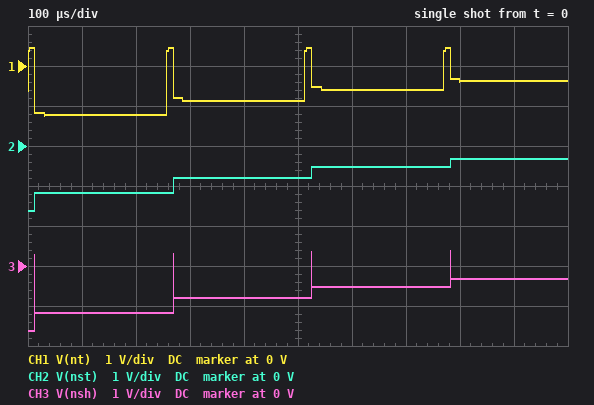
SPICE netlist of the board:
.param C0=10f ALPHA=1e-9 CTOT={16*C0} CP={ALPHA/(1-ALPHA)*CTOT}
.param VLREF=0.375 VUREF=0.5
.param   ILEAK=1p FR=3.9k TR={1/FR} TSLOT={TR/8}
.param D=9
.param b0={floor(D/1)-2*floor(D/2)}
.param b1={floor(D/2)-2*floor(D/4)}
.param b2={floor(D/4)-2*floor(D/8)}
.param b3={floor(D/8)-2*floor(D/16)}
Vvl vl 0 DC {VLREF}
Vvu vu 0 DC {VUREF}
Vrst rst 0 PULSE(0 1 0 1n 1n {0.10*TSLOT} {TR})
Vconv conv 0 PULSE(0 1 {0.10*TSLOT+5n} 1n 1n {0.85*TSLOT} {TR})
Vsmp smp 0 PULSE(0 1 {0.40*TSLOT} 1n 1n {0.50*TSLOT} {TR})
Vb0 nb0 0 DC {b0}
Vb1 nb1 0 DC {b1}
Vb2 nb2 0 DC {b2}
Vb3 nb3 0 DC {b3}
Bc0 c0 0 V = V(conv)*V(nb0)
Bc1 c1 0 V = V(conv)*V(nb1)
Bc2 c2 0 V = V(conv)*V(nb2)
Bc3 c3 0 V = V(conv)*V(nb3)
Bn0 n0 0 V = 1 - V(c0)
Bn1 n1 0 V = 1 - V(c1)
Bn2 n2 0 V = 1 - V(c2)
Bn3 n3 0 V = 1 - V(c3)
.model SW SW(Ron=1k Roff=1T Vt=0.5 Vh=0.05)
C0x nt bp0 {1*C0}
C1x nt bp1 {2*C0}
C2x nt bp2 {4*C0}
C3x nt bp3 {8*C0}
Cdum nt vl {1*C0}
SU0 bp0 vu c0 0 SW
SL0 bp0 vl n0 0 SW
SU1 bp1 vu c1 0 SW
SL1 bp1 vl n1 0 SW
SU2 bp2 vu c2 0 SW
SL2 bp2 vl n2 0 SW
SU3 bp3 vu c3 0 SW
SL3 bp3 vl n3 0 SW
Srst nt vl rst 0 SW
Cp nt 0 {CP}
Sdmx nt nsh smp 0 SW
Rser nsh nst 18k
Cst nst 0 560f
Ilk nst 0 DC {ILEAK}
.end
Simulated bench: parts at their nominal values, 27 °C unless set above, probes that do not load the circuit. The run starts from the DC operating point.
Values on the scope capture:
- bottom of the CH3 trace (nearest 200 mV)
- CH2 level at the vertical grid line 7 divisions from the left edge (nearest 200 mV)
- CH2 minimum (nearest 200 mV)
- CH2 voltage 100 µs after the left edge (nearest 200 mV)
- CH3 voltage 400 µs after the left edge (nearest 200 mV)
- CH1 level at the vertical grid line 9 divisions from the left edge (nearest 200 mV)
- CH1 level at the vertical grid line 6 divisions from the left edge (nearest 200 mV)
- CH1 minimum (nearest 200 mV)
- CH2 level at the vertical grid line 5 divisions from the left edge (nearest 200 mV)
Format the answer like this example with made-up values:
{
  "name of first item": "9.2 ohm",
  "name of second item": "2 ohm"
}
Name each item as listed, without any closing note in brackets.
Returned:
{
  "bottom of the CH3 trace": "-1.6 V",
  "CH2 level at the vertical grid line 7 divisions from the left edge": "-600 mV",
  "CH2 minimum": "-1.6 V",
  "CH2 voltage 100 µs after the left edge": "-1.2 V",
  "CH3 voltage 400 µs after the left edge": "-800 mV",
  "CH1 level at the vertical grid line 9 divisions from the left edge": "-400 mV",
  "CH1 level at the vertical grid line 6 divisions from the left edge": "-600 mV",
  "CH1 minimum": "-1.2 V",
  "CH2 level at the vertical grid line 5 divisions from the left edge": "-800 mV"
}
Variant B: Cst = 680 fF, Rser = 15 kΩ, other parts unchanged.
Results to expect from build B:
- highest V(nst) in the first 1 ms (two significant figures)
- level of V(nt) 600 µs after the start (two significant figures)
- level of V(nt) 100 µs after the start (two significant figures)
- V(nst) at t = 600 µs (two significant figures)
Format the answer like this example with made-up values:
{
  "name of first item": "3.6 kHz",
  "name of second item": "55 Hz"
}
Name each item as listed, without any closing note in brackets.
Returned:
{
  "highest V(nst) in the first 1 ms": "-440 mV",
  "level of V(nt) 600 µs after the start": "-720 mV",
  "level of V(nt) 100 µs after the start": "-1.3 V",
  "V(nst) at t = 600 µs": "-650 mV"
}
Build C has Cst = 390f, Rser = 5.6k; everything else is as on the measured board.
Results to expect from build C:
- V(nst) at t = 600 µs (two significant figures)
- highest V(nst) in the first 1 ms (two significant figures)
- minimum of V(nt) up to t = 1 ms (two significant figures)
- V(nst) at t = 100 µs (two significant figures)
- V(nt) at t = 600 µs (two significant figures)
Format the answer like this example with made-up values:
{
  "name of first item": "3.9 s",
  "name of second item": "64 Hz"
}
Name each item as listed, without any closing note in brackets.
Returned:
{
  "V(nst) at t = 600 µs": "-290 mV",
  "highest V(nst) in the first 1 ms": "-79 mV",
  "minimum of V(nt) up to t = 1 ms": "-1.1 V",
  "V(nst) at t = 100 µs": "-1.0 V",
  "V(nt) at t = 600 µs": "-360 mV"
}
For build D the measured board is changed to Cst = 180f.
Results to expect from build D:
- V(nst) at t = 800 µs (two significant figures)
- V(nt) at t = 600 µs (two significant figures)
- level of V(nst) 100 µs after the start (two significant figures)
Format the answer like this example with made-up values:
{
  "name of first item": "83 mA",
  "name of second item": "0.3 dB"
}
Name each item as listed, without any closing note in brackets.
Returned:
{
  "V(nst) at t = 800 µs": "280 mV",
  "V(nt) at t = 600 µs": "67 mV",
  "level of V(nst) 100 µs after the start": "-650 mV"
}
